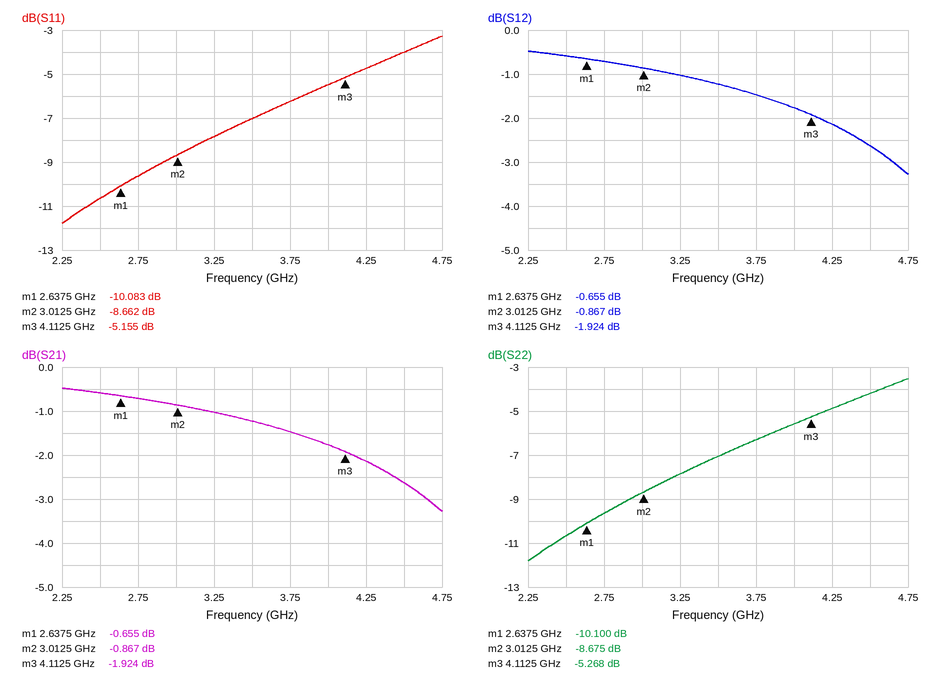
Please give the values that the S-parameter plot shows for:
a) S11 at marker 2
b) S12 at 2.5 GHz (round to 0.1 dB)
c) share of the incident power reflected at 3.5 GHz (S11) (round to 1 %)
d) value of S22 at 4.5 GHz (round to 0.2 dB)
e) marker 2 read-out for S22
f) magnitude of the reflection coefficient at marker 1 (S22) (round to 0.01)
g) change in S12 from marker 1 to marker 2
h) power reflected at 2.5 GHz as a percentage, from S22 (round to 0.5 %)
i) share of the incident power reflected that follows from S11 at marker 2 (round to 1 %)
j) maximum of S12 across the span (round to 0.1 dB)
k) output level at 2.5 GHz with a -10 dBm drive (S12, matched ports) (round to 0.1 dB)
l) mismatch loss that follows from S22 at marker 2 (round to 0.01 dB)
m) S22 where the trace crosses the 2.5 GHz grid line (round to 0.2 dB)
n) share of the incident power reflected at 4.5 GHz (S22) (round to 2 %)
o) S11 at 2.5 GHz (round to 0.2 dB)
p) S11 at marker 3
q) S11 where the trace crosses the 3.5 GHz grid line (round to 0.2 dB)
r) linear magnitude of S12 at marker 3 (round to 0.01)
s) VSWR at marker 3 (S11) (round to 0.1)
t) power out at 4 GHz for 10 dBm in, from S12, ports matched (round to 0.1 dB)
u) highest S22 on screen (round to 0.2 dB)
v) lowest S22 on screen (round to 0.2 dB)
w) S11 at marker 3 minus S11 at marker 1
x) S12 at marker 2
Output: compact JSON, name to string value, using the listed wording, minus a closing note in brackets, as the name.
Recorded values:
{"S11 at marker 2": "-8.662 dB", "S12 at 2.5 GHz": "-0.6 dB", "share of the incident power reflected at 3.5 GHz (S11)": "20 %", "value of S22 at 4.5 GHz": "-4.2 dB", "marker 2 read-out for S22": "-8.675 dB", "magnitude of the reflection coefficient at marker 1 (S22)": "0.31", "change in S12 from marker 1 to marker 2": "-0.212 dB", "power reflected at 2.5 GHz as a percentage, from S22": "8.5 %", "share of the incident power reflected that follows from S11 at marker 2": "14 %", "maximum of S12 across the span": "-0.5 dB", "output level at 2.5 GHz with a -10 dBm drive (S12, matched ports)": "-10.6 dBm", "mismatch loss that follows from S22 at marker 2": "0.63 dB", "S22 where the trace crosses the 2.5 GHz grid line": "-10.6 dB", "share of the incident power reflected at 4.5 GHz (S22)": "38 %", "S11 at 2.5 GHz": "-10.6 dB", "S11 at marker 3": "-5.155 dB", "S11 where the trace crosses the 3.5 GHz grid line": "-7.0 dB", "linear magnitude of S12 at marker 3": "0.80", "VSWR at marker 3 (S11)": "3.5", "power out at 4 GHz for 10 dBm in, from S12, ports matched": "8.2 dBm", "highest S22 on screen": "-3.6 dB", "lowest S22 on screen": "-11.8 dB", "S11 at marker 3 minus S11 at marker 1": "4.928 dB", "S12 at marker 2": "-0.867 dB"}
